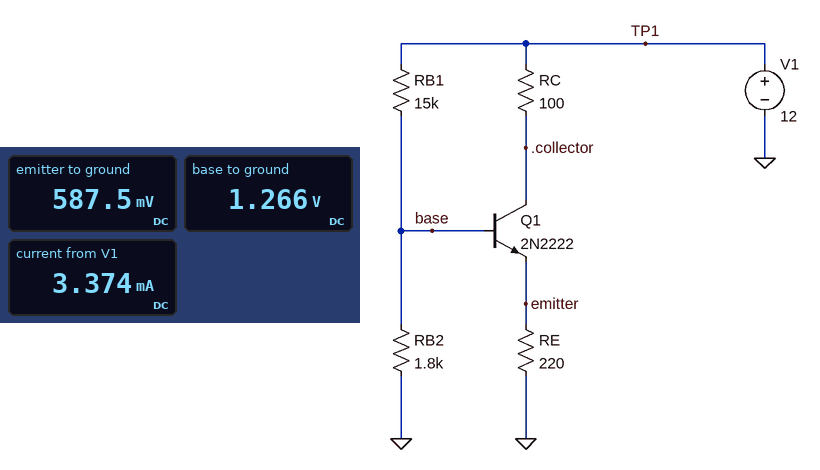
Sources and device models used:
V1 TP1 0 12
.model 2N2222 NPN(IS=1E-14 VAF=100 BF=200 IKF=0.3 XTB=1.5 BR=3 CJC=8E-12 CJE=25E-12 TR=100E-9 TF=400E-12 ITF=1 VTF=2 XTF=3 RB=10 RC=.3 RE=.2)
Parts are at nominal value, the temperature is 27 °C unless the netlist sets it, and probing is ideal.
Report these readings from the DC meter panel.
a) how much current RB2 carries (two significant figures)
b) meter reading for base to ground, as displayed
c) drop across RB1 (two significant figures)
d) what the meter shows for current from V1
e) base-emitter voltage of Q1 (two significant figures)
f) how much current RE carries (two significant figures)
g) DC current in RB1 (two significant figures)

700 µA
1.266 V
11 V
3.374 mA
680 mV
2.7 mA
720 µA
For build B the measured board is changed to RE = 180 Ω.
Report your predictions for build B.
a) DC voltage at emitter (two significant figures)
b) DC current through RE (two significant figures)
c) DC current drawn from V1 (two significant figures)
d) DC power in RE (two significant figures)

580 mV
3.2 mA
3.9 mA
1.9 mW
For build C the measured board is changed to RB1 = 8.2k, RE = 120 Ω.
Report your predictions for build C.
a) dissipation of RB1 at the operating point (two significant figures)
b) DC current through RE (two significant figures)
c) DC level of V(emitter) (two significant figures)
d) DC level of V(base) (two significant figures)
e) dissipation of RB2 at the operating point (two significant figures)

12 mW
11 mA
1.4 V
2.1 V
2.4 mW
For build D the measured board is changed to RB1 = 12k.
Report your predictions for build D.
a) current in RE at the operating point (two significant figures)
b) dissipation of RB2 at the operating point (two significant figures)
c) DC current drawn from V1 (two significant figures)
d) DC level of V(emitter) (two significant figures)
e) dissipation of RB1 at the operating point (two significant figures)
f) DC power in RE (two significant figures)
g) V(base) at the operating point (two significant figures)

3.9 mA
1.3 mW
4.7 mA
850 mV
9.1 mW
3.3 mW
1.5 V
